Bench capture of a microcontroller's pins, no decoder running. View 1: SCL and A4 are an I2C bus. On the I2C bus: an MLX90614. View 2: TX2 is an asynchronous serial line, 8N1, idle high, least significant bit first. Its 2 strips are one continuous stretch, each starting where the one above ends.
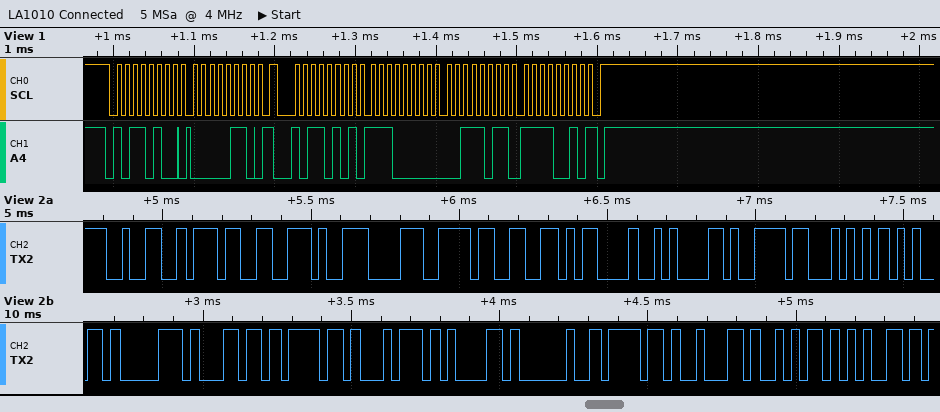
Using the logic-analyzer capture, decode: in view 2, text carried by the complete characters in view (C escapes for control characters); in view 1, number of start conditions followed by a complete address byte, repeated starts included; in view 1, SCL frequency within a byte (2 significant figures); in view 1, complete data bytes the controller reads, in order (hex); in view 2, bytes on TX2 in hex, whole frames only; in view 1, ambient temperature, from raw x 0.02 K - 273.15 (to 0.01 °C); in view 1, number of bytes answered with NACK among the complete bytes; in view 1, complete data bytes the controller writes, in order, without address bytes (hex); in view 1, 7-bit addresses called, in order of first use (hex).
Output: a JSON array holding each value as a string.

["\"27.83\\r\\nyTeplota obje\"", "2", "100 kHz", "E0 3B F2", "32 37 2E 38 33 0D 0A 79 54 65 70 6C 6F 74 61 20 6F 62 6A 65", "33.41 °C", "1", "06", "0x5A"]
